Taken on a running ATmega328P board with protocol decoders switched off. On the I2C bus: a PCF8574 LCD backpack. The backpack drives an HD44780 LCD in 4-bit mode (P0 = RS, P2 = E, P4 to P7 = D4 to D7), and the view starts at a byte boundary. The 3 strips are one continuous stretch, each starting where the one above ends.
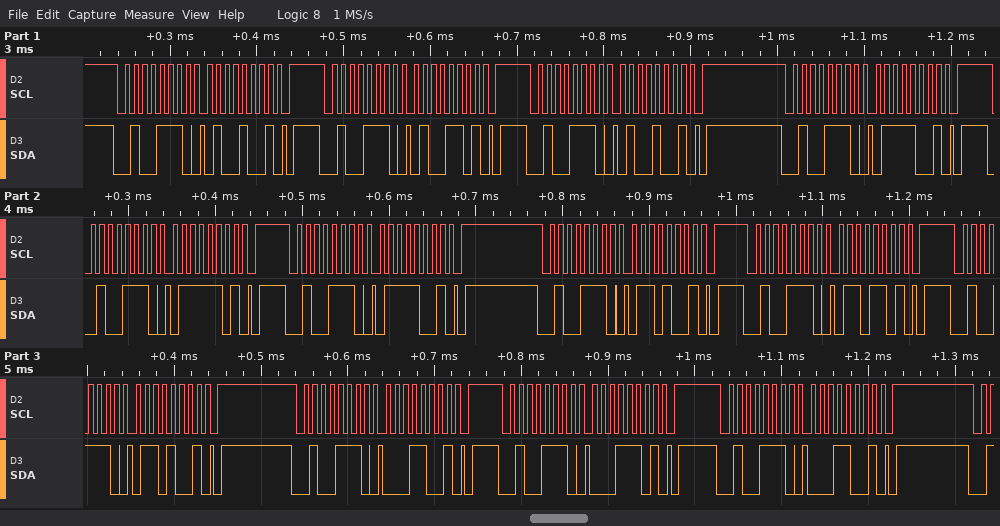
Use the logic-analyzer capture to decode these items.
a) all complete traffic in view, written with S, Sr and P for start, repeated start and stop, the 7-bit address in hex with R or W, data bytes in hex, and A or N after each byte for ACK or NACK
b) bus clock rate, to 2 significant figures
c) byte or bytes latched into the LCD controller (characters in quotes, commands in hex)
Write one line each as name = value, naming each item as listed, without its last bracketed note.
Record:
all complete traffic in view, written with S, Sr and P for start, repeated start and stop, the 7-bit address in hex with R or W, data bytes in hex, and A or N after each byte for ACK or NACK = S 27W A 49 A P S 27W A 4D A P S 27W A 49 A P S 27W A 79 A P S 27W A 7D A P S 27W A 79 A P S 27W A 69 A P S 27W A 6D A P S 27W A 69 A P S 27W A 19 A P S 27W A 1D A P S 27W A 19 A P
bus clock rate, to 2 significant figures = 100 kHz
byte or bytes latched into the LCD controller = 'G' 'a'
